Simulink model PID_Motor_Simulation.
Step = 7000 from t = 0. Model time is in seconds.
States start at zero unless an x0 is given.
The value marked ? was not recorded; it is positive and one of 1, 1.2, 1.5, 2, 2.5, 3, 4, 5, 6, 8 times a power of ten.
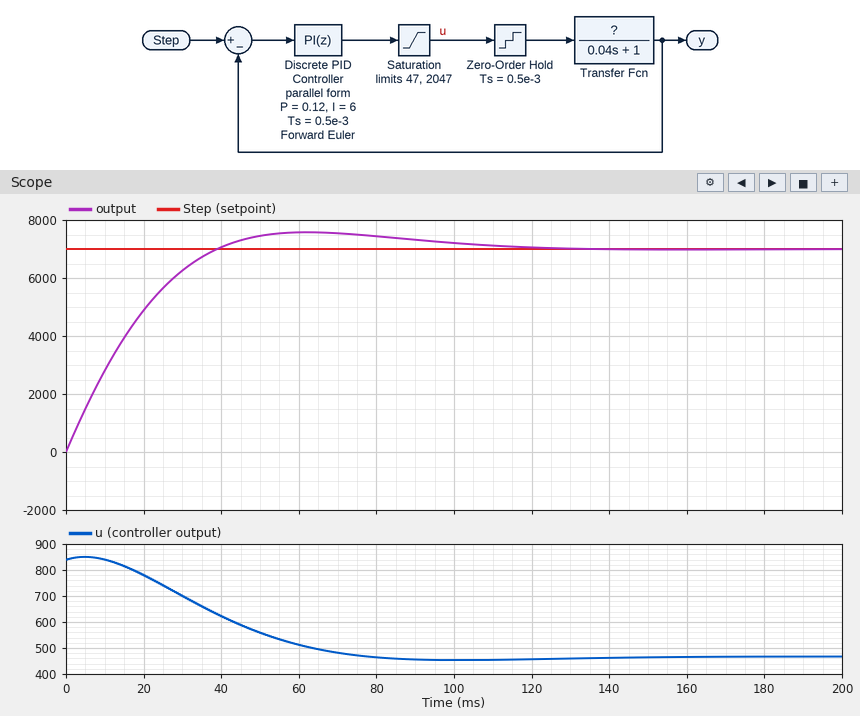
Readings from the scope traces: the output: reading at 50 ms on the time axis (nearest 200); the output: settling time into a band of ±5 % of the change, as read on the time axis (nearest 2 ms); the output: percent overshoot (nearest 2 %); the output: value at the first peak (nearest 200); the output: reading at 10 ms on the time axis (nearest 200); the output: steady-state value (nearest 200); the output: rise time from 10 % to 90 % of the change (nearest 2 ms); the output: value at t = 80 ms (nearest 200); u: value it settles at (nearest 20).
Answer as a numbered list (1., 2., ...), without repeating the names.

1. 7400
2. 88 ms
3. 8 %
4. 7600
5. 2800
6. 7000
7. 28 ms
8. 7400
9. 460
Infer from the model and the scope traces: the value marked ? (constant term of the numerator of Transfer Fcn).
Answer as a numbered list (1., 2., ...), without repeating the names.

1. 15
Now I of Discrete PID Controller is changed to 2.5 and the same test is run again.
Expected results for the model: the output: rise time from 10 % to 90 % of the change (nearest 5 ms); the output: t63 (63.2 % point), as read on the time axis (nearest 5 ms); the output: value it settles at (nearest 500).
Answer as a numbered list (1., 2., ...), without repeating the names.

1. 60 ms
2. 25 ms
3. 7000
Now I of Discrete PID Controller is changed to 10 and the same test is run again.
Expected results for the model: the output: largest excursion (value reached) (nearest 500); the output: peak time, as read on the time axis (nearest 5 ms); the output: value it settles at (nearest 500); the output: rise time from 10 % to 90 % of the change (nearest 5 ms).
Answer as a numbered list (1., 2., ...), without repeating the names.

1. 8000
2. 45 ms
3. 7000
4. 20 ms
